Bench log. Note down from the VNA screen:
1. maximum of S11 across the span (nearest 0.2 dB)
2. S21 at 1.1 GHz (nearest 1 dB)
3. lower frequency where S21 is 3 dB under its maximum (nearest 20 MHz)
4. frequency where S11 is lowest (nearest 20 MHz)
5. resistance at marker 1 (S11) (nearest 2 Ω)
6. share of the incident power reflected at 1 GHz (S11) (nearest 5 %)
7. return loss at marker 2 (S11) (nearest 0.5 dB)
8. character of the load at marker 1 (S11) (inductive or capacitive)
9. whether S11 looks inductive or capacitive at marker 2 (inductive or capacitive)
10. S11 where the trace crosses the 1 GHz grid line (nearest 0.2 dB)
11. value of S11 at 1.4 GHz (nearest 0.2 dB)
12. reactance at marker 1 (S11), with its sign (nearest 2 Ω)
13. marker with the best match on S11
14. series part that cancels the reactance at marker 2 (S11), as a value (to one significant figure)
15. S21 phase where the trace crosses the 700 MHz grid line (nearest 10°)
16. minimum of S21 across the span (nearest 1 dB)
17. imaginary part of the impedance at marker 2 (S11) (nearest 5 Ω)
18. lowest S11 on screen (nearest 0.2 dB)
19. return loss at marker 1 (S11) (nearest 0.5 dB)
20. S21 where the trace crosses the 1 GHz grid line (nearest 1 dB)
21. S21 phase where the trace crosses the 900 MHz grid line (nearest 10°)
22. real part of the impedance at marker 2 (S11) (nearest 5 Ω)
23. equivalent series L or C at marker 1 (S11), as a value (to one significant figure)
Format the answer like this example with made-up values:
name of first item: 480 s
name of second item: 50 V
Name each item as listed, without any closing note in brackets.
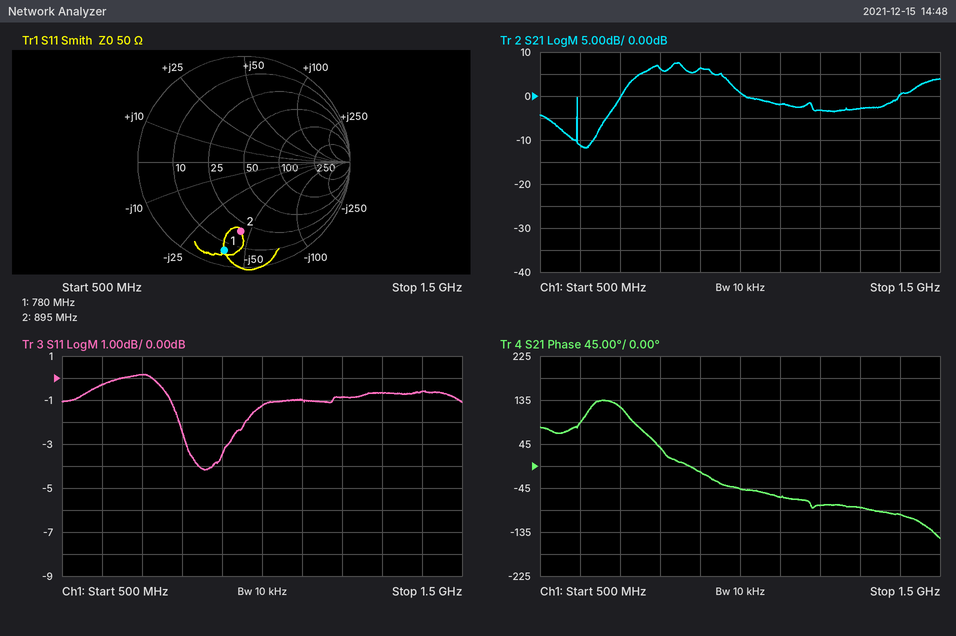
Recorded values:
maximum of S11 across the span: 0.2 dB
S21 at 1.1 GHz: -2 dB
lower frequency where S21 is 3 dB under its maximum: 740 MHz
frequency where S11 is lowest: 860 MHz
resistance at marker 1 (S11): 6 Ω
share of the incident power reflected at 1 GHz (S11): 75 %
return loss at marker 2 (S11): 3.5 dB
character of the load at marker 1 (S11): capacitive
whether S11 looks inductive or capacitive at marker 2: capacitive
S11 where the trace crosses the 1 GHz grid line: -1.2 dB
value of S11 at 1.4 GHz: -0.6 dB
reactance at marker 1 (S11), with its sign: -40 Ω
marker with the best match on S11: marker 2
series part that cancels the reactance at marker 2 (S11), as a value: 8 nH
S21 phase where the trace crosses the 700 MHz grid line: 120°
minimum of S21 across the span: -12 dB
imaginary part of the impedance at marker 2 (S11): -45 Ω
lowest S11 on screen: -4.2 dB
return loss at marker 1 (S11): 1.5 dB
S21 where the trace crosses the 1 GHz grid line: 1 dB
S21 phase where the trace crosses the 900 MHz grid line: -10°
real part of the impedance at marker 2 (S11): 20 Ω
equivalent series L or C at marker 1 (S11), as a value: 5 pF
